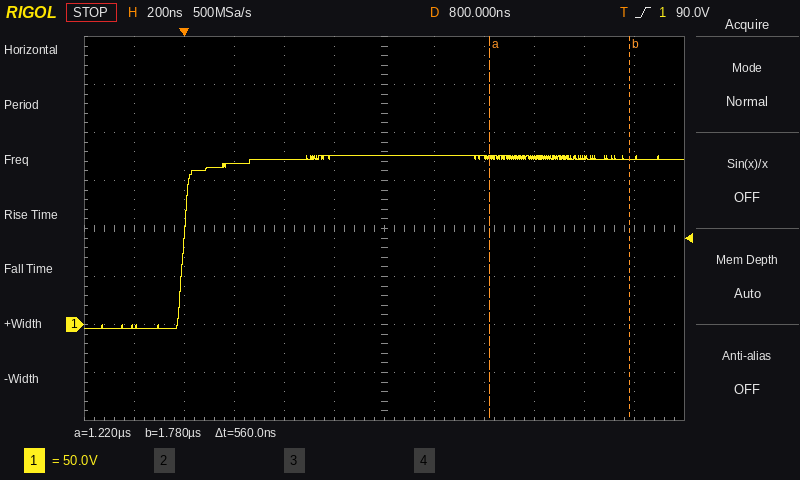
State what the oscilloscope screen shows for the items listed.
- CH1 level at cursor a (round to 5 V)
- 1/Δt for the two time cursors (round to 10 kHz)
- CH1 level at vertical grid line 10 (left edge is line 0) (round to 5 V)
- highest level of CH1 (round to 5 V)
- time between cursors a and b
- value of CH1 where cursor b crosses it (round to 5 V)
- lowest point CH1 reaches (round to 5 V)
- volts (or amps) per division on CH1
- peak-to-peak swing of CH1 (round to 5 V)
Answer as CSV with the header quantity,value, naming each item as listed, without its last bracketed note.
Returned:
quantity,value
CH1 level at cursor a,175 V
1/Δt for the two time cursors,1.79 MHz
CH1 level at vertical grid line 10 (left edge is line 0),175 V
highest level of CH1,175 V
time between cursors a and b,560 ns
value of CH1 where cursor b crosses it,170 V
lowest point CH1 reaches,-5 V
volts (or amps) per division on CH1,50 V
peak-to-peak swing of CH1,180 V
